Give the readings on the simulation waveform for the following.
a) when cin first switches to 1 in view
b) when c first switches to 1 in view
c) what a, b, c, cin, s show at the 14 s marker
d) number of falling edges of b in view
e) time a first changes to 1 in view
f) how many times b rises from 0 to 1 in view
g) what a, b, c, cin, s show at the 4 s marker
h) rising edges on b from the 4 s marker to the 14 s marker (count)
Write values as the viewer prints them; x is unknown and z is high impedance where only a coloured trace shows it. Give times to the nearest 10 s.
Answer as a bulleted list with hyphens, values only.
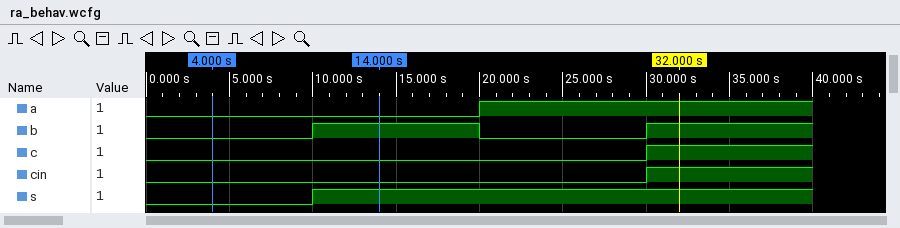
- 30 s
- 30 s
- a=0, b=1, c=0, cin=0, s=1
- 1
- 20 s
- 2
- a=0, b=0, c=0, cin=0, s=0
- 1
